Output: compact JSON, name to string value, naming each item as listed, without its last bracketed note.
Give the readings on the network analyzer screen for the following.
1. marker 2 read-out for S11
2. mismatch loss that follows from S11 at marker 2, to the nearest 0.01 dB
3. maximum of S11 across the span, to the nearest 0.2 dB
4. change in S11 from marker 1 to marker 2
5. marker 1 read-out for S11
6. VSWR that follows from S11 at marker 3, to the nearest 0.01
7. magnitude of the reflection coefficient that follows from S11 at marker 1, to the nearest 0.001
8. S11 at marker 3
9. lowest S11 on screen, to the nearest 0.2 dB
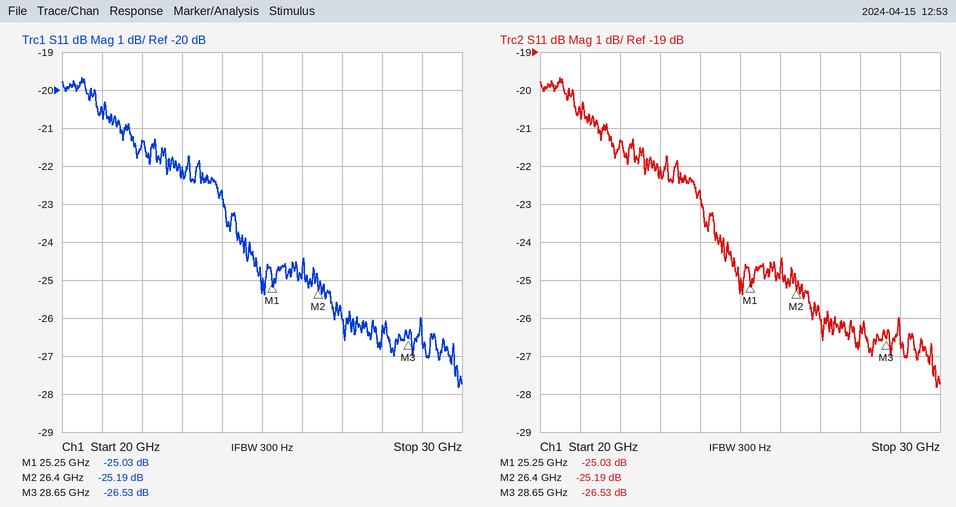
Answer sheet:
{"marker 2 read-out for S11": "-25.19 dB", "mismatch loss that follows from S11 at marker 2, to the nearest 0.01 dB": "0.01 dB", "maximum of S11 across the span, to the nearest 0.2 dB": "-19.6 dB", "change in S11 from marker 1 to marker 2": "-0.16 dB", "marker 1 read-out for S11": "-25.03 dB", "VSWR that follows from S11 at marker 3, to the nearest 0.01": "1.10", "magnitude of the reflection coefficient that follows from S11 at marker 1, to the nearest 0.001": "0.056", "S11 at marker 3": "-26.53 dB", "lowest S11 on screen, to the nearest 0.2 dB": "-27.8 dB"}
